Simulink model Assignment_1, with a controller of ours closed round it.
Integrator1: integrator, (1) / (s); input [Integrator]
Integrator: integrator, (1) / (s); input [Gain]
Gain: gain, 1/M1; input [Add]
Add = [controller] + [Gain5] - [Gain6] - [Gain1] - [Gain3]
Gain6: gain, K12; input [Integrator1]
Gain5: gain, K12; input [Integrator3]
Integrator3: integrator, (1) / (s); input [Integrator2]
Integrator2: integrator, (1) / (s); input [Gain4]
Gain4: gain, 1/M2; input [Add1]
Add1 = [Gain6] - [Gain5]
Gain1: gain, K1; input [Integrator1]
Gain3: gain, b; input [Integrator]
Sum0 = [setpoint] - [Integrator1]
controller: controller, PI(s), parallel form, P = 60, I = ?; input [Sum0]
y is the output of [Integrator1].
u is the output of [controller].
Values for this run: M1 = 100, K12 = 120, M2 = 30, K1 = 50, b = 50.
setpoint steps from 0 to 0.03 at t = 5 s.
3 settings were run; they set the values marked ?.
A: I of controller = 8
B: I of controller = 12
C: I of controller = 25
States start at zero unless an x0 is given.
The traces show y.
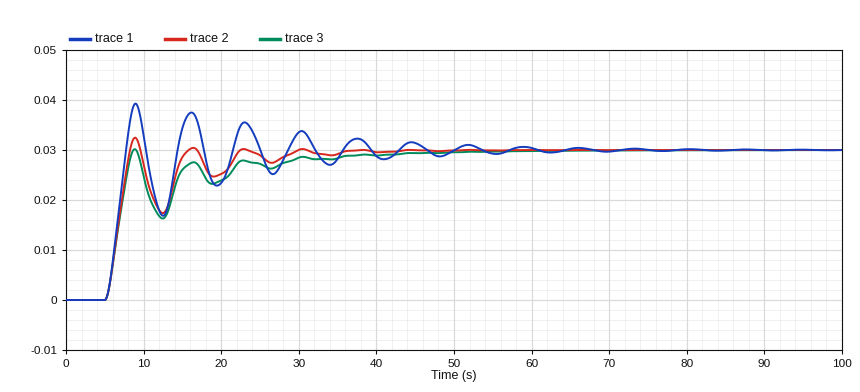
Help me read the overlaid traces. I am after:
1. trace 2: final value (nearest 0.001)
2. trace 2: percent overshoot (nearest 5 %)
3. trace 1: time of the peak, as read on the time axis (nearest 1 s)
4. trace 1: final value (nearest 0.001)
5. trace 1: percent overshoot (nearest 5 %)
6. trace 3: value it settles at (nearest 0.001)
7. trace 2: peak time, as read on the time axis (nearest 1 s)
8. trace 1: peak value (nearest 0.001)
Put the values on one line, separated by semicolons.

0.030; 10 %; 9 s; 0.030; 30 %; 0.030; 9 s; 0.039
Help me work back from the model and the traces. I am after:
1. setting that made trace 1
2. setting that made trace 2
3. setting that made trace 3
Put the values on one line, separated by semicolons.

C; B; A
